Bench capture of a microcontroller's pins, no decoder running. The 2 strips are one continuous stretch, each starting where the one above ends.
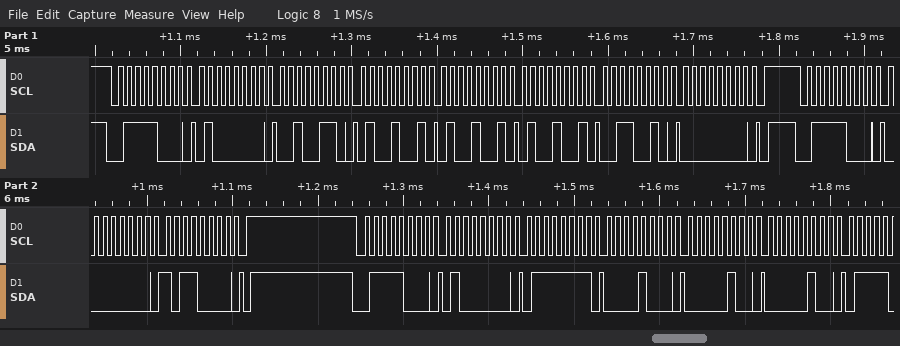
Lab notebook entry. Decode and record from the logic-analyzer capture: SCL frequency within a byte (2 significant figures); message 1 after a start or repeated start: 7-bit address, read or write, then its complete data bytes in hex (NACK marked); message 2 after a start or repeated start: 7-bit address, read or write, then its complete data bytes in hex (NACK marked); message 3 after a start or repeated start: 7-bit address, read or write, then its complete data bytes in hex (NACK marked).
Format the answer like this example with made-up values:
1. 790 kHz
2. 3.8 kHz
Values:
1. 100 kHz
2. 0x3C write: 40 26 49 49 49 32 00
3. 0x3C write: 00 B0
4. 0x3C write: 40 7F 08 04 04
